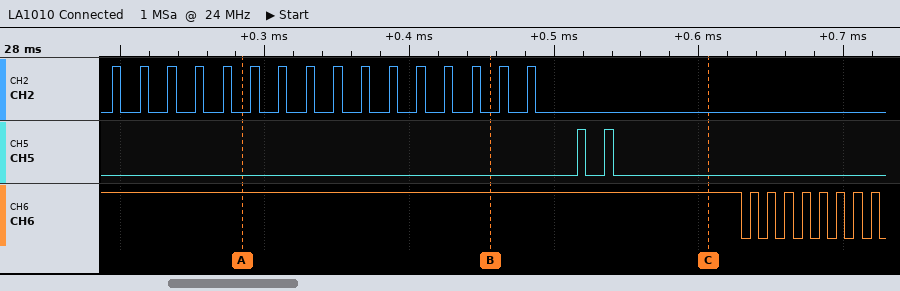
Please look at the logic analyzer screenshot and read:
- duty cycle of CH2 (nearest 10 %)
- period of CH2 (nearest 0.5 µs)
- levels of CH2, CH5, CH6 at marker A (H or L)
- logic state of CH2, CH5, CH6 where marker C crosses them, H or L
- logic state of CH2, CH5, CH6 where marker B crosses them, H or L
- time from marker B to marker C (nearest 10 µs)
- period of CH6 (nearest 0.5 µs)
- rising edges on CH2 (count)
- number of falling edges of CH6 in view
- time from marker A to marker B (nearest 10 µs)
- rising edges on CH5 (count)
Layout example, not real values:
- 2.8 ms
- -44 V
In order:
- 30 %
- 19 µs
- CH2=L, CH5=L, CH6=H
- CH2=L, CH5=L, CH6=H
- CH2=L, CH5=L, CH6=H
- 150 µs
- 12 µs
- 16
- 9
- 170 µs
- 2
